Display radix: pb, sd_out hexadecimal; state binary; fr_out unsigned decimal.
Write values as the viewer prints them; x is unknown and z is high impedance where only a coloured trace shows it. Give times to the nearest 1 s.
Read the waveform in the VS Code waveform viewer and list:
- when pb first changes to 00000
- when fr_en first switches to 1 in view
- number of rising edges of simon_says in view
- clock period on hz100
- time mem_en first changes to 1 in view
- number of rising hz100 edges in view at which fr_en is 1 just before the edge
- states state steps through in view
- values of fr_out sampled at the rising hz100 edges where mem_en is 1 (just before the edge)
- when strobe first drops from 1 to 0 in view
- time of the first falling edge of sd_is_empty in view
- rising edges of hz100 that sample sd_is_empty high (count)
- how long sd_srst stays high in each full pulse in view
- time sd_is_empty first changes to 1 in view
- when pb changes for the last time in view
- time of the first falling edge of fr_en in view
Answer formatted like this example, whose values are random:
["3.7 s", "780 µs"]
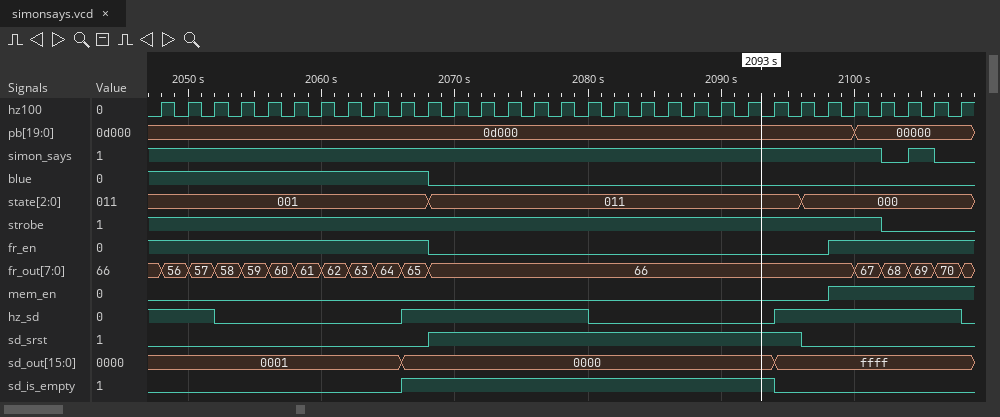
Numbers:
["2100 s", "2098 s", "1", "2 s", "2098 s", "16", "001, 011, 000", "66, 67, 68, 69, 70", "2102 s", "2094 s", "14", "28 s", "2066 s", "2100 s", "2068 s"]
